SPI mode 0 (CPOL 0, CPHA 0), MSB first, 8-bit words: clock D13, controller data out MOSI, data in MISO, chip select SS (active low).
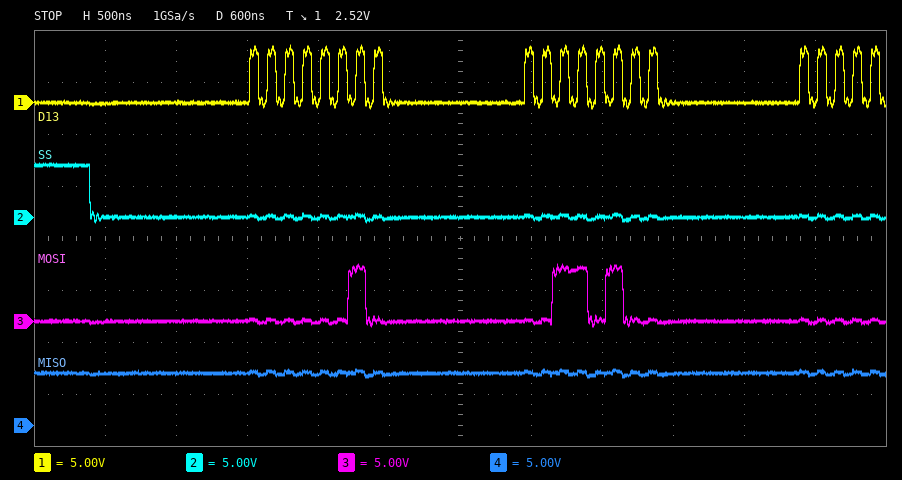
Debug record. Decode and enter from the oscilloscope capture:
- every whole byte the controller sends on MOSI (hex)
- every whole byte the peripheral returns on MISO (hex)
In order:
02 34
FF FF
